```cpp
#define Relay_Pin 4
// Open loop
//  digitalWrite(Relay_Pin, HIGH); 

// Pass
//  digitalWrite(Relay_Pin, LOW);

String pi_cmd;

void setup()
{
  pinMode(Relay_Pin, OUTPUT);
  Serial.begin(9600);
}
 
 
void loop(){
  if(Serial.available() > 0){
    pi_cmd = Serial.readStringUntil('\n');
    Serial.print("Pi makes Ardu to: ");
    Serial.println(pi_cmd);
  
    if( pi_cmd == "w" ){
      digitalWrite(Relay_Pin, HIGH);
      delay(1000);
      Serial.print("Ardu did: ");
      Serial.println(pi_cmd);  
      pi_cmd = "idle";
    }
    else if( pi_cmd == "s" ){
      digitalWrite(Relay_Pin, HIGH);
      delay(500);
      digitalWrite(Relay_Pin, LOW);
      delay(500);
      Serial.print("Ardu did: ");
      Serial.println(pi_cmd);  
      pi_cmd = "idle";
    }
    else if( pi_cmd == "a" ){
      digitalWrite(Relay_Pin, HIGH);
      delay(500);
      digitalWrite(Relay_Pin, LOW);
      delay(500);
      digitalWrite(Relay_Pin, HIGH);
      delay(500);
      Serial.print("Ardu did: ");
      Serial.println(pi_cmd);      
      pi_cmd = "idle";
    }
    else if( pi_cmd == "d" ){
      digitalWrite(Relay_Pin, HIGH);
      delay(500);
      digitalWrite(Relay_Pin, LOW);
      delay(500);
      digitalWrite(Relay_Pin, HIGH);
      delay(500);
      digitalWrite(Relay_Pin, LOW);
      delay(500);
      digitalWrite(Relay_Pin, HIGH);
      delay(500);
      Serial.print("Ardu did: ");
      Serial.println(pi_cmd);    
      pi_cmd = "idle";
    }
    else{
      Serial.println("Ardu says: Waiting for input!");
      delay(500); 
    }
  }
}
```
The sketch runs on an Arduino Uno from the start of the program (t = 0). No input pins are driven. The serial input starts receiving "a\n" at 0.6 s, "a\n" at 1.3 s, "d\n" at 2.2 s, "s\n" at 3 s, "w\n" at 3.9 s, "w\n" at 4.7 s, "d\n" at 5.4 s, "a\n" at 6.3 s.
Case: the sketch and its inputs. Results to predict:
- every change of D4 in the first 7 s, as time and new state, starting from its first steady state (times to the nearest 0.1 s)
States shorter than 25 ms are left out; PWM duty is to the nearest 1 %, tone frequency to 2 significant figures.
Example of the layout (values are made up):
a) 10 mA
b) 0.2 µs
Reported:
a) 0 s low; 0.6 s high; 1.1 s low; 1.6 s high; 2.6 s low; 3.1 s high; 4.1 s low; 4.6 s high; 5.1 s low; 5.6 s high; 6.6 s low
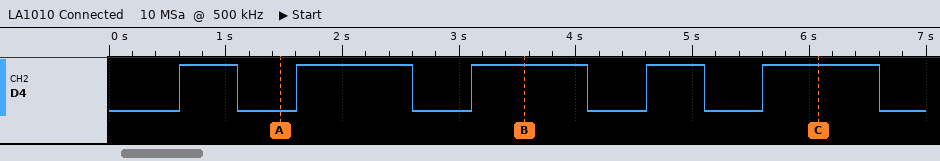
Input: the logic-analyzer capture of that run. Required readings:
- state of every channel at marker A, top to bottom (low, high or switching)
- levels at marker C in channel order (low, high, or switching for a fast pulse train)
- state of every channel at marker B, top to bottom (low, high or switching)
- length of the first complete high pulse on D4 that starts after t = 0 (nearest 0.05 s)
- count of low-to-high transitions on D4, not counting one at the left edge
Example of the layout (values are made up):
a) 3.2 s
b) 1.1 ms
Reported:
a) D4 low
b) D4 high
c) D4 high
d) 0.50 s
e) 5
